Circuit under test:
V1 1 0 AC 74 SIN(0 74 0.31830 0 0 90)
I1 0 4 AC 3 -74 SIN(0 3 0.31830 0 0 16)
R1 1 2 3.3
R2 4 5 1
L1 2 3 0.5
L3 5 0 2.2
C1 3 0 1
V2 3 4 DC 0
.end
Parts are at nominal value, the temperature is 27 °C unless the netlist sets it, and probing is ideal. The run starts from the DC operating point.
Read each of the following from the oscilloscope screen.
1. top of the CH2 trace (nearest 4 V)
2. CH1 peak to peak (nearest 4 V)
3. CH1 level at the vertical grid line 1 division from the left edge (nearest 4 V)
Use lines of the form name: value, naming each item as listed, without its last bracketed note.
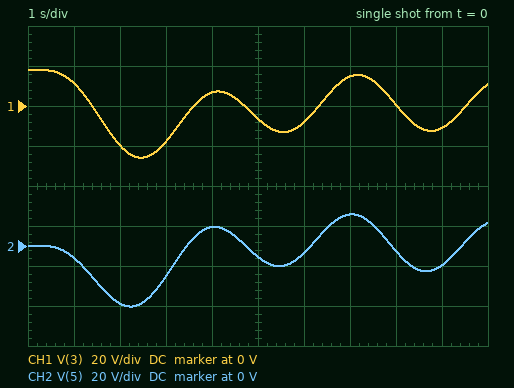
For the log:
top of the CH2 trace: 16 V
CH1 peak to peak: 44 V
CH1 level at the vertical grid line 1 division from the left edge: 12 V
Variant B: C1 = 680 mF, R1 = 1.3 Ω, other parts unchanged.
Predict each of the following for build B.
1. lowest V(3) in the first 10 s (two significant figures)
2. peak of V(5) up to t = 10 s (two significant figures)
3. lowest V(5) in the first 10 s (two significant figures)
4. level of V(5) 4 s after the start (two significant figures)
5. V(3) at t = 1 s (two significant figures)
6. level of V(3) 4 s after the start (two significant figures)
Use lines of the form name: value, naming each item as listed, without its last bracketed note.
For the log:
lowest V(3) in the first 10 s: -65 V
peak of V(5) up to t = 10 s: 52 V
lowest V(5) in the first 10 s: -70 V
level of V(5) 4 s after the start: 50 V
V(3) at t = 1 s: 16 V
level of V(3) 4 s after the start: 53 V
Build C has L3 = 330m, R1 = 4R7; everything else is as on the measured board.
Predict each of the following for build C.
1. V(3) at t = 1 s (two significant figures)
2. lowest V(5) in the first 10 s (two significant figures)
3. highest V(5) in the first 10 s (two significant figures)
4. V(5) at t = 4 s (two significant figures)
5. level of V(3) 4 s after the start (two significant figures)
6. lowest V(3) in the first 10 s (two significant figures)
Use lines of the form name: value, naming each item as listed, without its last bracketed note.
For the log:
V(3) at t = 1 s: 9.1 V
lowest V(5) in the first 10 s: -6.0 V
highest V(5) in the first 10 s: 5.4 V
V(5) at t = 4 s: 1.4 V
level of V(3) 4 s after the start: 9.2 V
lowest V(3) in the first 10 s: -10 V
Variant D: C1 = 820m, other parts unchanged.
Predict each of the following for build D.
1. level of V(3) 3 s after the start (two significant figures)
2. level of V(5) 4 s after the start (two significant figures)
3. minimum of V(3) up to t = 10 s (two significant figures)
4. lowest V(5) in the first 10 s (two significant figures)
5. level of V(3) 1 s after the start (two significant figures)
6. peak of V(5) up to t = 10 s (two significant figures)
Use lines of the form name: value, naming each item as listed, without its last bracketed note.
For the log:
level of V(3) 3 s after the start: -19 V
level of V(5) 4 s after the start: 16 V
minimum of V(3) up to t = 10 s: -31 V
lowest V(5) in the first 10 s: -34 V
level of V(3) 1 s after the start: 10 V
peak of V(5) up to t = 10 s: 18 V
